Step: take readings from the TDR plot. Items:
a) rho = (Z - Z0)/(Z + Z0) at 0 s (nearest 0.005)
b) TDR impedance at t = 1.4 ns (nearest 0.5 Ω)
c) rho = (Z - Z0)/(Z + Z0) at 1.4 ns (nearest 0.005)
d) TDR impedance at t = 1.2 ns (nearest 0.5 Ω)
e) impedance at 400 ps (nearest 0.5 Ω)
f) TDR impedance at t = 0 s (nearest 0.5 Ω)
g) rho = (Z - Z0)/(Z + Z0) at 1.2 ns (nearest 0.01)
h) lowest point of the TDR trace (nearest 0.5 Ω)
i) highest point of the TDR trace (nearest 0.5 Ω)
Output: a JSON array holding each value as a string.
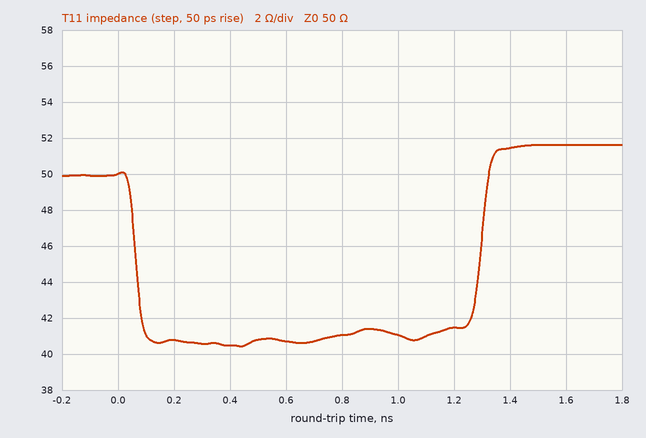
["0.000", "51.5 Ω", "+0.015", "41.5 Ω", "40.5 Ω", "50.0 Ω", "-0.09", "40.5 Ω", "51.5 Ω"]
